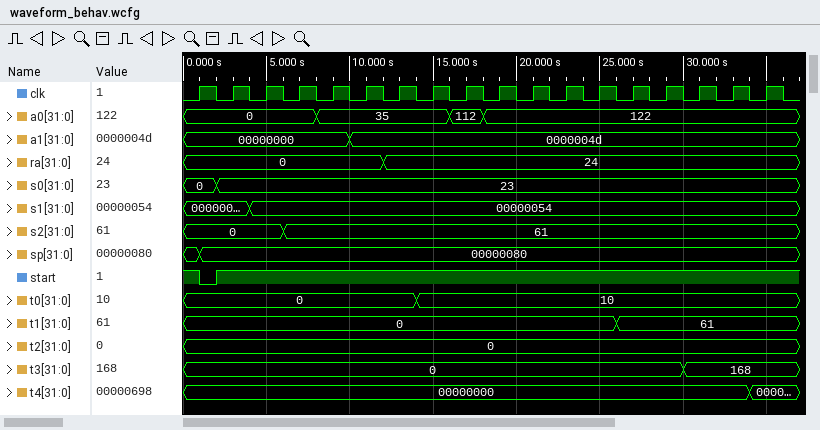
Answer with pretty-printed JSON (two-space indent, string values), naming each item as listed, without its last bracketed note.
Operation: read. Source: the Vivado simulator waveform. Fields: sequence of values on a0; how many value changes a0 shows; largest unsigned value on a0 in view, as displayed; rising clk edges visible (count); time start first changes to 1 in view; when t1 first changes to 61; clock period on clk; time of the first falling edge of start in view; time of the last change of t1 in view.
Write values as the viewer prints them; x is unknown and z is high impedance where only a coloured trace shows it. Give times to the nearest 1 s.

{
  "sequence of values on a0": "0, 35, 112, 122",
  "how many value changes a0 shows": "3",
  "largest unsigned value on a0 in view, as displayed": "122",
  "rising clk edges visible": "18",
  "time start first changes to 1 in view": "2 s",
  "when t1 first changes to 61": "26 s",
  "clock period on clk": "2 s",
  "time of the first falling edge of start in view": "1 s",
  "time of the last change of t1 in view": "26 s"
}
